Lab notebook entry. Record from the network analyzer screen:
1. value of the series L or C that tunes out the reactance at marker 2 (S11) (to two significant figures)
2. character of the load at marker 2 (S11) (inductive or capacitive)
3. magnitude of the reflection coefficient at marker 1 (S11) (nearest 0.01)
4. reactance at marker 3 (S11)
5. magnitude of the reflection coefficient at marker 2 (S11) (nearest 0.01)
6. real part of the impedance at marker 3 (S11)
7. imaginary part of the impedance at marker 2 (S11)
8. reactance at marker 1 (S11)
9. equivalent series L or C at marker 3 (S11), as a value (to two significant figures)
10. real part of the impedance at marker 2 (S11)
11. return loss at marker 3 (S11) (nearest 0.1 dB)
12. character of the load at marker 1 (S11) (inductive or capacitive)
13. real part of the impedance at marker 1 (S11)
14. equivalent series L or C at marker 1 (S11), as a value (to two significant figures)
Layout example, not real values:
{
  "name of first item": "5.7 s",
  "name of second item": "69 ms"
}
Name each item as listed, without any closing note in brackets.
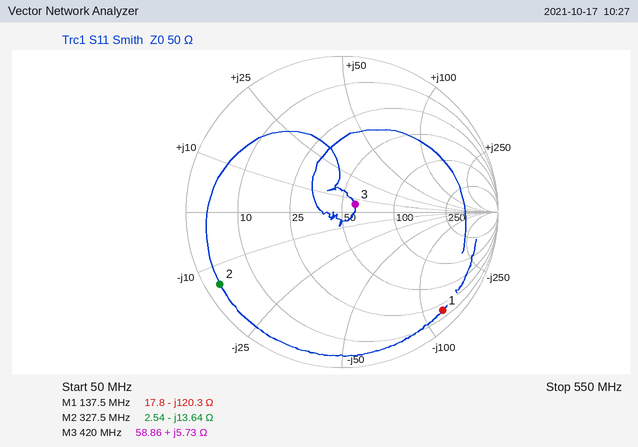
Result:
{
  "value of the series L or C that tunes out the reactance at marker 2 (S11)": "6.6 nH",
  "character of the load at marker 2 (S11)": "capacitive",
  "magnitude of the reflection coefficient at marker 1 (S11)": "0.90",
  "reactance at marker 3": "+5.73 Ω",
  "magnitude of the reflection coefficient at marker 2 (S11)": "0.91",
  "real part of the impedance at marker 3": "58.86 Ω",
  "imaginary part of the impedance at marker 2": "-13.64 Ω",
  "reactance at marker 1": "-120.3 Ω",
  "equivalent series L or C at marker 3 (S11), as a value": "2.2 nH",
  "real part of the impedance at marker 2": "2.54 Ω",
  "return loss at marker 3 (S11)": "20.3 dB",
  "character of the load at marker 1 (S11)": "capacitive",
  "real part of the impedance at marker 1": "17.8 Ω",
  "equivalent series L or C at marker 1 (S11), as a value": "9.6 pF"
}
